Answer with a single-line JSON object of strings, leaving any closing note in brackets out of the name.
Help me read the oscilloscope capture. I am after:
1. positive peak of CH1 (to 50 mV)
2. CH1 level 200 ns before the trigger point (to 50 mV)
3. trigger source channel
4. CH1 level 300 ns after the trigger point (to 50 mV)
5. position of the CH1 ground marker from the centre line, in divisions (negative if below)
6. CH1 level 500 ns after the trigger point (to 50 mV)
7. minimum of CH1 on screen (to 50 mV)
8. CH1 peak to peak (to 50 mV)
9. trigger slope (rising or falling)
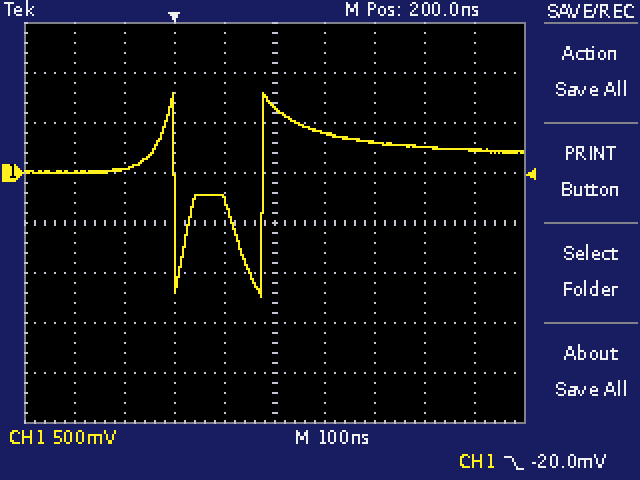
{"positive peak of CH1": "800 mV", "CH1 level 200 ns before the trigger point": "0 mV", "trigger source channel": "CH1", "CH1 level 300 ns after the trigger point": "400 mV", "position of the CH1 ground marker from the centre line, in divisions": "+1.0 div", "CH1 level 500 ns after the trigger point": "250 mV", "minimum of CH1 on screen": "-1.25 V", "CH1 peak to peak": "2.05 V", "trigger slope": "falling"}
